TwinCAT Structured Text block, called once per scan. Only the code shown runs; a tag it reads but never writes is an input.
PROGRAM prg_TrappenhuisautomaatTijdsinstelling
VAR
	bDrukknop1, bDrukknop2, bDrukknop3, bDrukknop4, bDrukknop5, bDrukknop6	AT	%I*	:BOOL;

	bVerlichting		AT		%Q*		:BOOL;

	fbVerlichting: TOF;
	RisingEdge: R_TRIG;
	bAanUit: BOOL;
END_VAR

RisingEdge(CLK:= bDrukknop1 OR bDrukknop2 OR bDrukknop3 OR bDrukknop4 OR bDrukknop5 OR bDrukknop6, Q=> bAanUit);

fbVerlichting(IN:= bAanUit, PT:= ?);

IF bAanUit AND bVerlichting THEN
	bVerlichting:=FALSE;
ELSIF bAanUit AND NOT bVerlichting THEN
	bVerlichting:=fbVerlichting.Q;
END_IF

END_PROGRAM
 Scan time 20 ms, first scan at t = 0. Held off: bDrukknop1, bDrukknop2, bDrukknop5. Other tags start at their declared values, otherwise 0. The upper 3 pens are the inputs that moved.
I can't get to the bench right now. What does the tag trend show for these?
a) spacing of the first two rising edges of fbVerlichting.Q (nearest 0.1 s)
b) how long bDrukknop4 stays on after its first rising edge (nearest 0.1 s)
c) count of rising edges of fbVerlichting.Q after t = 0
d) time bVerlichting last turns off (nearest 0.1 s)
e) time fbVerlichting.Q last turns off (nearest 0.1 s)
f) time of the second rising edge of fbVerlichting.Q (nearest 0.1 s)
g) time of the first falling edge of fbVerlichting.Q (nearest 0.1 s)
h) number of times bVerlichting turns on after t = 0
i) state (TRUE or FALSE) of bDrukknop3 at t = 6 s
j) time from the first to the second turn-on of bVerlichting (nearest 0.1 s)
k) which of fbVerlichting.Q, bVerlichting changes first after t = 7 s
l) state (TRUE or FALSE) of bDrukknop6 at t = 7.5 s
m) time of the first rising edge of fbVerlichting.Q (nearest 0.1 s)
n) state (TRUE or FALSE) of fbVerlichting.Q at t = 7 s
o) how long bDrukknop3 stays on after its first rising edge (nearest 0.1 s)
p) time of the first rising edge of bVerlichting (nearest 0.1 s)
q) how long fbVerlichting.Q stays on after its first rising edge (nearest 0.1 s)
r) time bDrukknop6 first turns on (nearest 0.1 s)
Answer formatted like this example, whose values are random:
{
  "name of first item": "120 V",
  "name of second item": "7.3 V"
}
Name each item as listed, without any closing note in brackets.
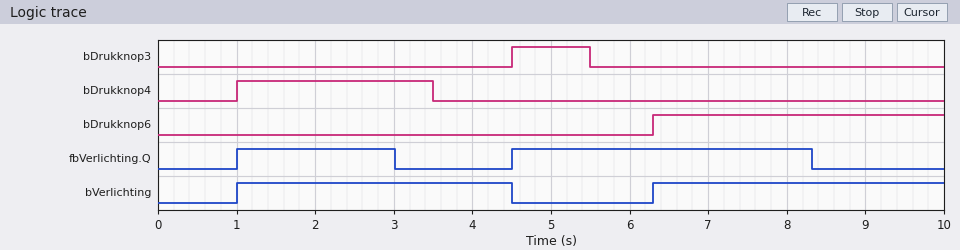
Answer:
{
  "spacing of the first two rising edges of fbVerlichting.Q": "3.5 s",
  "how long bDrukknop4 stays on after its first rising edge": "2.5 s",
  "count of rising edges of fbVerlichting.Q after t = 0": "2",
  "time bVerlichting last turns off": "4.5 s",
  "time fbVerlichting.Q last turns off": "8.3 s",
  "time of the second rising edge of fbVerlichting.Q": "4.5 s",
  "time of the first falling edge of fbVerlichting.Q": "3.0 s",
  "number of times bVerlichting turns on after t = 0": "2",
  "state (TRUE or FALSE) of bDrukknop3 at t = 6 s": "FALSE",
  "time from the first to the second turn-on of bVerlichting": "5.3 s",
  "which of fbVerlichting.Q, bVerlichting changes first after t = 7 s": "fbVerlichting.Q",
  "state (TRUE or FALSE) of bDrukknop6 at t = 7.5 s": "TRUE",
  "time of the first rising edge of fbVerlichting.Q": "1.0 s",
  "state (TRUE or FALSE) of fbVerlichting.Q at t = 7 s": "TRUE",
  "how long bDrukknop3 stays on after its first rising edge": "1.0 s",
  "time of the first rising edge of bVerlichting": "1.0 s",
  "how long fbVerlichting.Q stays on after its first rising edge": "2.0 s",
  "time bDrukknop6 first turns on": "6.3 s"
}
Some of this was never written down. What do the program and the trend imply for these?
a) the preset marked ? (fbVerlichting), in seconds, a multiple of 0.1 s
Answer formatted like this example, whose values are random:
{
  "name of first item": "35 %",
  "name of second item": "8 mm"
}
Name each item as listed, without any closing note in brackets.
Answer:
{
  "the preset marked ? (fbVerlichting), in seconds, a multiple of 0.1 s": "2.0 s"
}
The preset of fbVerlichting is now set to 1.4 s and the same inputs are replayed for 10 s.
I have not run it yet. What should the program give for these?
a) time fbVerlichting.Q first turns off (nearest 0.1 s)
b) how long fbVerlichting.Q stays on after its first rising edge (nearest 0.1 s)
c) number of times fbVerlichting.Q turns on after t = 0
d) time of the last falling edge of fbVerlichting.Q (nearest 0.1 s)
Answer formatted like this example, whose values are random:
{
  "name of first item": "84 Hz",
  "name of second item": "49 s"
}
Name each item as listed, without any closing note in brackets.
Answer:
{
  "time fbVerlichting.Q first turns off": "2.4 s",
  "how long fbVerlichting.Q stays on after its first rising edge": "1.4 s",
  "number of times fbVerlichting.Q turns on after t = 0": "3",
  "time of the last falling edge of fbVerlichting.Q": "7.7 s"
}
